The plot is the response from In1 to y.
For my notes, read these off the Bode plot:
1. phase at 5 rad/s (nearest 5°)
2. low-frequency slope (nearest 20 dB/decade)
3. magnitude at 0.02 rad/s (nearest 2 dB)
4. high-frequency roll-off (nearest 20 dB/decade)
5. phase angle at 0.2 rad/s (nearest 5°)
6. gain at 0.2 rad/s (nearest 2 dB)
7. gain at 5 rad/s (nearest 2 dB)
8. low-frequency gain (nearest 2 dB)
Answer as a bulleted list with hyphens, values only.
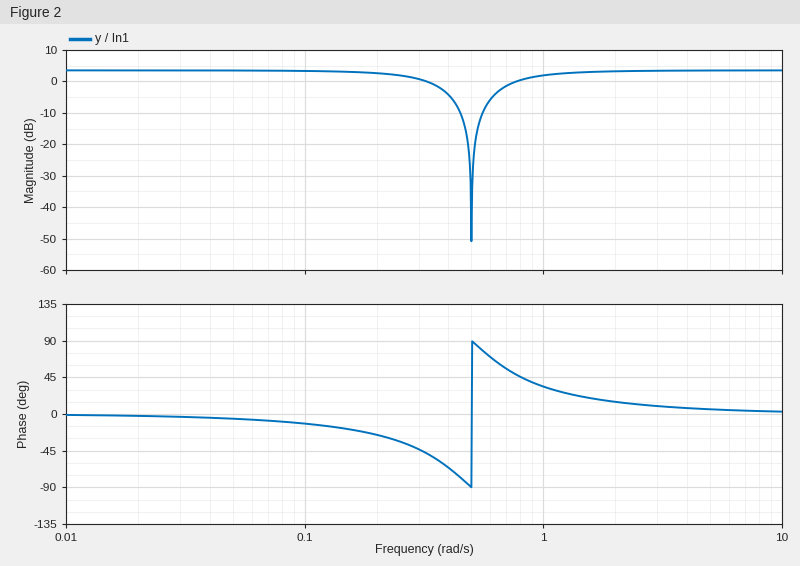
- 5°
- 0 dB/decade
- 4 dB
- 0 dB/decade
- -25°
- 2 dB
- 4 dB
- 4 dB
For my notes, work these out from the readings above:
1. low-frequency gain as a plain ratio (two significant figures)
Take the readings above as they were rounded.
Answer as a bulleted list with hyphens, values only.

- 1.6
